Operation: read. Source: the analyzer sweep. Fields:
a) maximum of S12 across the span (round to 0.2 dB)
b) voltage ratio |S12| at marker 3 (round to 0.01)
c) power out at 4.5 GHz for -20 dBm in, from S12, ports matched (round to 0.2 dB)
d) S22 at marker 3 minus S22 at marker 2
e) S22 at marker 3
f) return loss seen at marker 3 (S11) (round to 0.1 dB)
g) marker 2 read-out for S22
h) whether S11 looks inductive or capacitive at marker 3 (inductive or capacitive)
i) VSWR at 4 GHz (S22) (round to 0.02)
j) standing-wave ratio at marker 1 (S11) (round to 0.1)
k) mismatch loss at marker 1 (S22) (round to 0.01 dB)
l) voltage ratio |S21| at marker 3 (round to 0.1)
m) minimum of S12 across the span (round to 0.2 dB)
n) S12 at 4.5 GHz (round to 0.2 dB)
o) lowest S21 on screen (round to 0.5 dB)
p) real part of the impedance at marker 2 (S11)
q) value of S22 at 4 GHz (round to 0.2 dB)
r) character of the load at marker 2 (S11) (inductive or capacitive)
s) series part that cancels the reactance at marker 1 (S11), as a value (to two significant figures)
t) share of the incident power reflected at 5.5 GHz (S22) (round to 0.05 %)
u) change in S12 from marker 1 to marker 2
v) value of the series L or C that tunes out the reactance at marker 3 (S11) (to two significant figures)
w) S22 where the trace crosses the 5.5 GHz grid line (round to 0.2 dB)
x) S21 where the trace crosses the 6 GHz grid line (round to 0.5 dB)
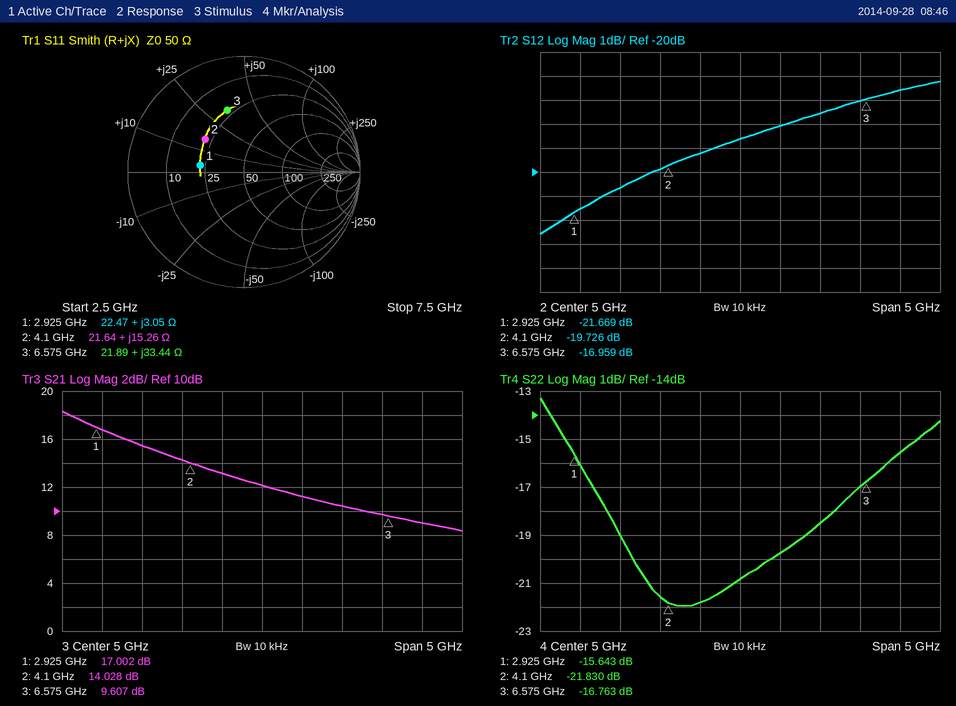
-16.2 dB
0.14
-39.2 dBm
5.067 dB
-16.763 dB
5.2 dB
-21.830 dB
inductive
1.18
2.2
0.12 dB
3.0
-22.6 dB
-19.2 dB
8.5 dB
21.64 Ω
-21.6 dB
inductive
18 pF
1.05 %
1.943 dB
720 fF
-19.8 dB
10.5 dB
